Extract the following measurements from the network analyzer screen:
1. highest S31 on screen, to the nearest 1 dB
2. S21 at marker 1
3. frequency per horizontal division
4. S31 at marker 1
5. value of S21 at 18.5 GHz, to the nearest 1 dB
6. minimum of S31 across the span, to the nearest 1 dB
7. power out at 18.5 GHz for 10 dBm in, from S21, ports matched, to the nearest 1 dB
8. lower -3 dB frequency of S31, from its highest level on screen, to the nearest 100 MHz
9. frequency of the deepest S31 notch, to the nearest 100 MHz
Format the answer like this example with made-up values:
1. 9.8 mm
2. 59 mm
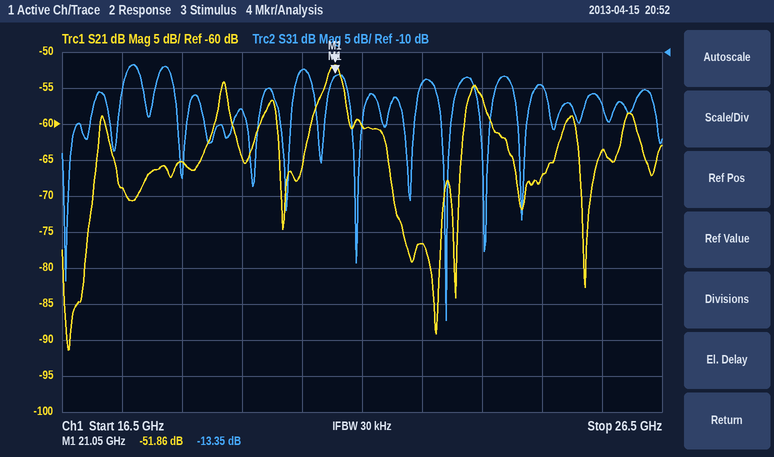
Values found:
1. -12 dB
2. -51.86 dB
3. 1 GHz
4. -13.35 dB
5. -65 dB
6. -47 dB
7. -55 dBm
8. 17.5 GHz
9. 22.9 GHz
